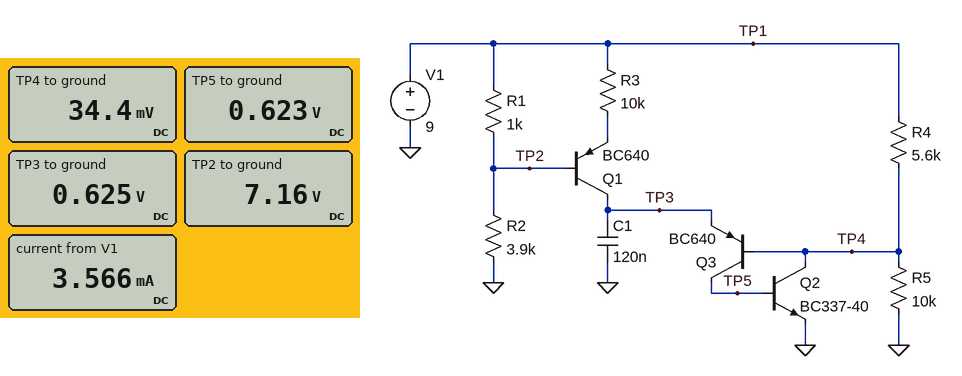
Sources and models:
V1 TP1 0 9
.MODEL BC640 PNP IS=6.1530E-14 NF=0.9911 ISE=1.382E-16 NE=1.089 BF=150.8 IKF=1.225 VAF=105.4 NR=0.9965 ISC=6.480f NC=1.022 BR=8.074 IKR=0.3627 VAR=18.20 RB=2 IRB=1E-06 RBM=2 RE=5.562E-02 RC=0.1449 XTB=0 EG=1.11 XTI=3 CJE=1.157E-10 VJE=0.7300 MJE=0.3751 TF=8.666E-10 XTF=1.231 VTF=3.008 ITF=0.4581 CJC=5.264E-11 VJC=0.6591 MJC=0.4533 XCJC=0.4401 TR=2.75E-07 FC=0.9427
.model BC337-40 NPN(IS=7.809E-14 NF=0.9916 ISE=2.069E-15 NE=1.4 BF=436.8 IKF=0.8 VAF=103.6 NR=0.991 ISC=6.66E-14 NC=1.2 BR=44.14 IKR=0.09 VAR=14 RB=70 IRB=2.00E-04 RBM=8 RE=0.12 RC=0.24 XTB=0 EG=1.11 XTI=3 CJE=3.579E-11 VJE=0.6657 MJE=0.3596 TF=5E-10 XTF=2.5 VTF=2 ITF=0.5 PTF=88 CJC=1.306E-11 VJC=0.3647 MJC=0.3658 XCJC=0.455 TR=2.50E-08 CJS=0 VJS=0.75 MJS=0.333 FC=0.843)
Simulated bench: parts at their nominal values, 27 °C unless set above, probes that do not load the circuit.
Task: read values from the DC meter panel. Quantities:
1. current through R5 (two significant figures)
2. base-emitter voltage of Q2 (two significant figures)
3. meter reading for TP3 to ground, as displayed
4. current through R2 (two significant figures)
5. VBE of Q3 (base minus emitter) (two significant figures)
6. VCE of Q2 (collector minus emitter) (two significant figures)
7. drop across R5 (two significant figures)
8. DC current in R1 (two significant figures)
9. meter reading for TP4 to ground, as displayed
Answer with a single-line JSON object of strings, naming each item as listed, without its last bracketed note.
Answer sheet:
{"current through R5": "3.4 µA", "base-emitter voltage of Q2": "620 mV", "meter reading for TP3 to ground, as displayed": "0.625 V", "current through R2": "1.8 mA", "VBE of Q3 (base minus emitter)": "-590 mV", "VCE of Q2 (collector minus emitter)": "34 mV", "drop across R5": "34 mV", "DC current in R1": "1.8 mA", "meter reading for TP4 to ground, as displayed": "34.4 mV"}
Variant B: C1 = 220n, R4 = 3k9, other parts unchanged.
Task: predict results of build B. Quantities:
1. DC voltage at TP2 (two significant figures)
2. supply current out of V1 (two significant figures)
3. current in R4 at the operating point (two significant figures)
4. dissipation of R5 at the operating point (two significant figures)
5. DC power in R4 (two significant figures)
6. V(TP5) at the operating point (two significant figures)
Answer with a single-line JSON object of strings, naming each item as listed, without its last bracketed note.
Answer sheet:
{"DC voltage at TP2": "7.2 V", "supply current out of V1": "4.3 mA", "current in R4 at the operating point": "2.3 mA", "dissipation of R5 at the operating point": "170 nW", "DC power in R4": "21 mW", "V(TP5) at the operating point": "630 mV"}
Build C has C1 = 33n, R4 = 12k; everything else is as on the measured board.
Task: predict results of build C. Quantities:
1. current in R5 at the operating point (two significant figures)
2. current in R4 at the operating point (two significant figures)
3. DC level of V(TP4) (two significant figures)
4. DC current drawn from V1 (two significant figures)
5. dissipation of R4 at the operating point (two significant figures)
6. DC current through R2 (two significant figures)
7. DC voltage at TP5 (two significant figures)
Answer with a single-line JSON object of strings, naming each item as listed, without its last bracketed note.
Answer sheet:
{"current in R5 at the operating point": "2.2 µA", "current in R4 at the operating point": "750 µA", "DC level of V(TP4)": "22 mV", "DC current drawn from V1": "2.7 mA", "dissipation of R4 at the operating point": "6.7 mW", "DC current through R2": "1.8 mA", "DC voltage at TP5": "610 mV"}
